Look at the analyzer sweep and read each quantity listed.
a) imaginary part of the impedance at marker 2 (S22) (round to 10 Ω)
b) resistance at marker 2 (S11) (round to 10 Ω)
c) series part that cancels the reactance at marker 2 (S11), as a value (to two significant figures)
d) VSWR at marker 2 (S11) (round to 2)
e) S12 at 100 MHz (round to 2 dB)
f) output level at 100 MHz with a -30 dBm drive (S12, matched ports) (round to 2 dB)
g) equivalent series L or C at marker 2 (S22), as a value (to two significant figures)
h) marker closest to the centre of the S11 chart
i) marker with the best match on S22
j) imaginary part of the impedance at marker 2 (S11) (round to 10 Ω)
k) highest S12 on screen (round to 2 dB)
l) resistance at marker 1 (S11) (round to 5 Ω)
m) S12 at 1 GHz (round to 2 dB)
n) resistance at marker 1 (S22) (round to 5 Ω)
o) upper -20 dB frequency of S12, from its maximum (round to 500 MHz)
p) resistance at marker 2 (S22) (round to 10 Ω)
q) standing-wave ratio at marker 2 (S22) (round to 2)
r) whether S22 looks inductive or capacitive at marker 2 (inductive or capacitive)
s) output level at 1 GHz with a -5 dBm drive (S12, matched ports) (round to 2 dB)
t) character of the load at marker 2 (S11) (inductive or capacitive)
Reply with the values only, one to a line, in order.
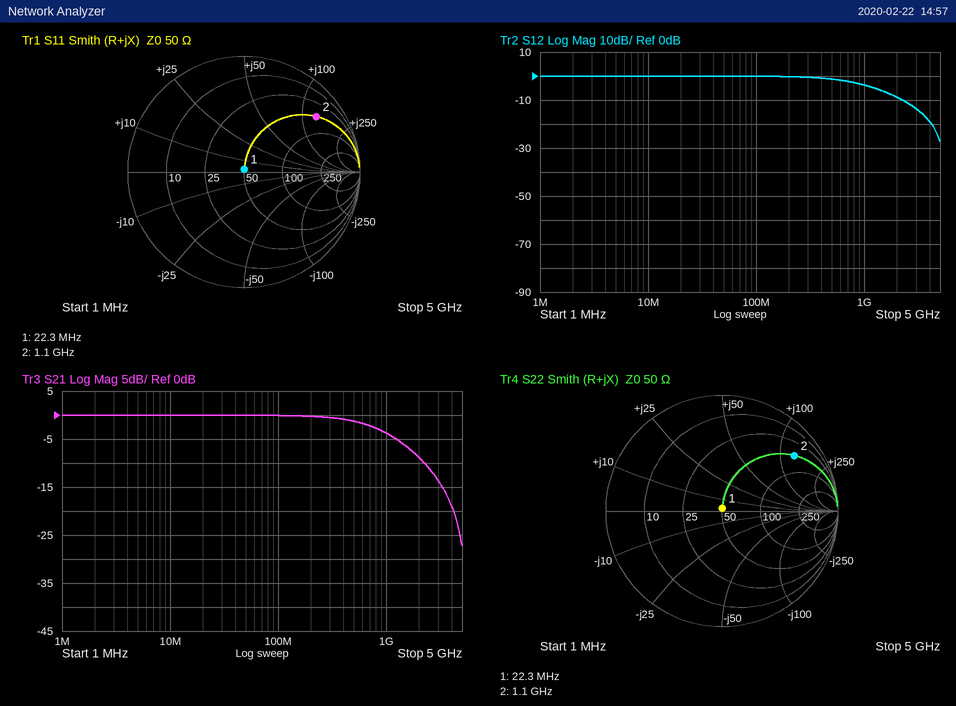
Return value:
+130 Ω
50 Ω
1.1 pF
8
0 dB
-30 dBm
19 nH
marker 1
marker 1
+130 Ω
0 dB
50 Ω
-4 dB
50 Ω
4.0 GHz
50 Ω
8
inductive
-8 dBm
inductive
